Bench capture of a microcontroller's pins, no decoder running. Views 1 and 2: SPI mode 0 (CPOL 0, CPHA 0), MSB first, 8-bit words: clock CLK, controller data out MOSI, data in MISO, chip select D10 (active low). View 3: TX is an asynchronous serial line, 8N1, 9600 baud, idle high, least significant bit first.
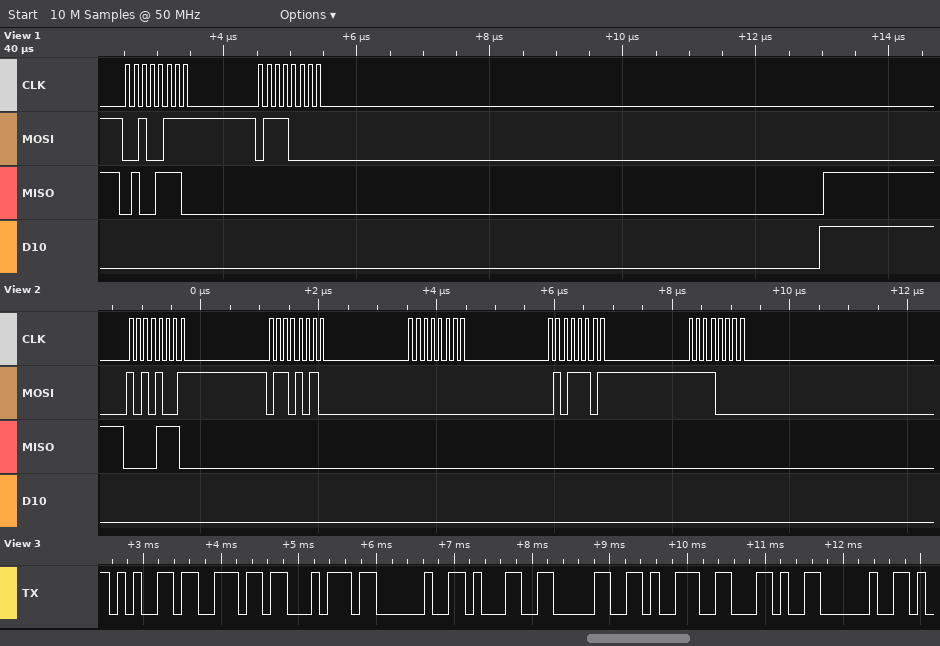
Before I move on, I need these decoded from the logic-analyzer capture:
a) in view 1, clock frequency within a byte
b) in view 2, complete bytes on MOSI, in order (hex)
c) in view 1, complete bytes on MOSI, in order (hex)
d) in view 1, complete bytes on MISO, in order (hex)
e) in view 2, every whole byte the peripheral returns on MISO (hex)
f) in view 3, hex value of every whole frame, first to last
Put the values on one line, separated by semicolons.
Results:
8 MHz; A9 6A 00 5D F0; 27 70; 4E 00; 0E 00 00 00 00; 0x65 0x6E 0x74 0x20 0x31 0x30 0x39 0x2C 0x20
